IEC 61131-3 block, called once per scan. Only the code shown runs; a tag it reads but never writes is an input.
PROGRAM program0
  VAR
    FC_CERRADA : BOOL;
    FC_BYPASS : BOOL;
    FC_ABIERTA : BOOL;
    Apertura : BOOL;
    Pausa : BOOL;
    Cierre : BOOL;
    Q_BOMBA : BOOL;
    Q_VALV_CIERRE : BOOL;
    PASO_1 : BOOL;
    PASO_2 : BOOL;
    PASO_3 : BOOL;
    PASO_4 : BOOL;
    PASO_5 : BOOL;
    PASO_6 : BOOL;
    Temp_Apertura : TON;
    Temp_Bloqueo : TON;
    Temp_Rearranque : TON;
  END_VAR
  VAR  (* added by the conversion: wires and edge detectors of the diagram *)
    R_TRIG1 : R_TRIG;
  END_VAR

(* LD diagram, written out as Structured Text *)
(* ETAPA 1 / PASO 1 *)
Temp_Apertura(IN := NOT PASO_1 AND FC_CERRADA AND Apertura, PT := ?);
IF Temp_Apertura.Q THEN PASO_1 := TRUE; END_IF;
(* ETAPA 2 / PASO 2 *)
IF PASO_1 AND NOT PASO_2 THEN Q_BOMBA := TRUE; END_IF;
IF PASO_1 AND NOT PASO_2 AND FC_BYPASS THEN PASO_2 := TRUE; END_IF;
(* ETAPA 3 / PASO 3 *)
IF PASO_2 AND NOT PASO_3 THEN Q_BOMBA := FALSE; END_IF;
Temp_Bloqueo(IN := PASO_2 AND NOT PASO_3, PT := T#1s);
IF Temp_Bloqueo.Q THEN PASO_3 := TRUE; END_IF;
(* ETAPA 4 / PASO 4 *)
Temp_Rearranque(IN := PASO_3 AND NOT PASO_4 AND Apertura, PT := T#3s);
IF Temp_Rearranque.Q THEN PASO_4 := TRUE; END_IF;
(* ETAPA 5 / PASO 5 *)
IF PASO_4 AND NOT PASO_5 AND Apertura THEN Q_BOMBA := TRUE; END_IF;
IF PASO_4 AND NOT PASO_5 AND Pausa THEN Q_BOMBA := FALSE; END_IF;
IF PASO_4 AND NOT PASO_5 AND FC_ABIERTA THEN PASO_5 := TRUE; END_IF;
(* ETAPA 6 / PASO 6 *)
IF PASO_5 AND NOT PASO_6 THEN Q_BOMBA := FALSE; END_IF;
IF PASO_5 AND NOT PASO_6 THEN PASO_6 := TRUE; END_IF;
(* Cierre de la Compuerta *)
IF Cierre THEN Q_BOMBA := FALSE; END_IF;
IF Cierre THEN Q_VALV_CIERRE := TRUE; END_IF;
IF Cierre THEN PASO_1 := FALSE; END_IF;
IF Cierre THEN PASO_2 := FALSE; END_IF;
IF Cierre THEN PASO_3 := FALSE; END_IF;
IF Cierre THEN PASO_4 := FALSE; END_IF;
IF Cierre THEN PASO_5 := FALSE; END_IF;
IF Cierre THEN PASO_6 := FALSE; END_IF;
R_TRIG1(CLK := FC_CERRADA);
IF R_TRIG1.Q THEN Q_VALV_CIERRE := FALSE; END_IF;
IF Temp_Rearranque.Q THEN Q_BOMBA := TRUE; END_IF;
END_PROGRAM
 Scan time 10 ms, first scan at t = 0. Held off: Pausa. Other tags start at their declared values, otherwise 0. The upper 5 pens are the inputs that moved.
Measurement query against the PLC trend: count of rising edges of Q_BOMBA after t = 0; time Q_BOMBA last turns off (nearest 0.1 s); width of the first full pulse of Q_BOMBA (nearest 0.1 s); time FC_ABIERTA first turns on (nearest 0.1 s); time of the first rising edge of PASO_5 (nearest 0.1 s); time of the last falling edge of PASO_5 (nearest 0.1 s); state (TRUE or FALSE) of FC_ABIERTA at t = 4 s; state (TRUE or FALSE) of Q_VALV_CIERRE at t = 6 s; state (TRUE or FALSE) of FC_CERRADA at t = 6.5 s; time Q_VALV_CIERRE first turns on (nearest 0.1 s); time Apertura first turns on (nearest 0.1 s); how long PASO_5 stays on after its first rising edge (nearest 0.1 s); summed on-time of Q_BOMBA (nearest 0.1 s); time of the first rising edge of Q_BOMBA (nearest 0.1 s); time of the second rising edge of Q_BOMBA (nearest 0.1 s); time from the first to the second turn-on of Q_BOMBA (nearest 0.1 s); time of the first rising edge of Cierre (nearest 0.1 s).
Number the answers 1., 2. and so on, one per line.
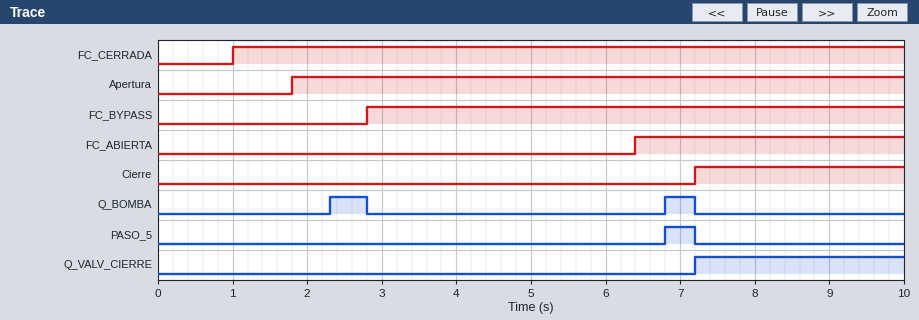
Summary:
1. 2
2. 7.2 s
3. 0.5 s
4. 6.4 s
5. 6.8 s
6. 7.2 s
7. FALSE
8. FALSE
9. TRUE
10. 7.2 s
11. 1.8 s
12. 0.4 s
13. 0.9 s
14. 2.3 s
15. 6.8 s
16. 4.5 s
17. 7.2 s
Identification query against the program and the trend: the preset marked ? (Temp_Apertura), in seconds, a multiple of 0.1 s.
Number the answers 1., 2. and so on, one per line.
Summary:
1. 0.5 s
